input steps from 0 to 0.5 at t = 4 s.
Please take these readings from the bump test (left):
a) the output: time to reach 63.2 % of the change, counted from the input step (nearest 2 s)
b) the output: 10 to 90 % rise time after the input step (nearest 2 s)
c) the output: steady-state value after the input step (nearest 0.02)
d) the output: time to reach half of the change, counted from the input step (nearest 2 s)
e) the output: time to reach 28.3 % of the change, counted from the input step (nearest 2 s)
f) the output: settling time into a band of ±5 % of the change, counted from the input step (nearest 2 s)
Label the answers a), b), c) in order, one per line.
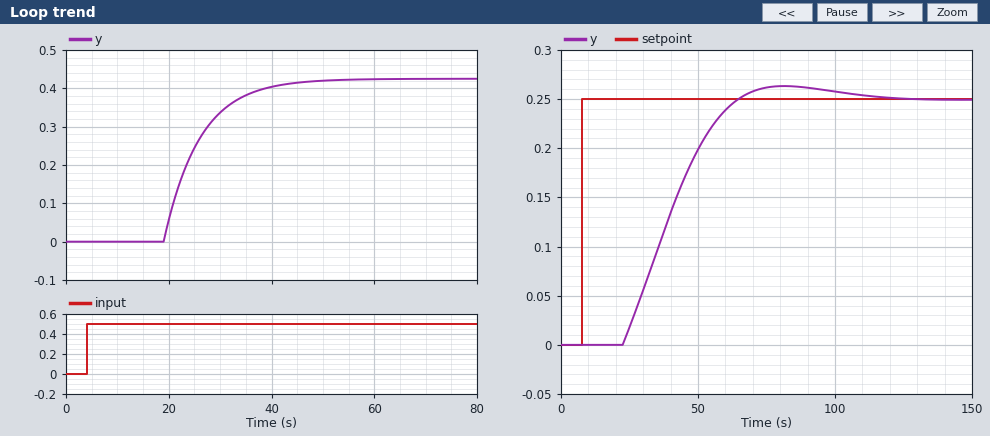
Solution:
a) 22 s
b) 16 s
c) 0.42
d) 20 s
e) 18 s
f) 36 s
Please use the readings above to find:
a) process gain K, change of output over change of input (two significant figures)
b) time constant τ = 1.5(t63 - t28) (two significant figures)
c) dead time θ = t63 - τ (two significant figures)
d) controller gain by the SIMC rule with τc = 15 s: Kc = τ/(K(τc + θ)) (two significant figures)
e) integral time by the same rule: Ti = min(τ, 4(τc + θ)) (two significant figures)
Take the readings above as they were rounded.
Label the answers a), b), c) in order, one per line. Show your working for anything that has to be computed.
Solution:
a) (0.42 - 0) / 0.5 = 0.84
b) 1.5 × (22 - 18) = 6.0 s
c) 22 - 6 = 16 s
d) 6 / (0.84 × (15 + 16)) = 0.23
e) min(6, 4 × (15 + 16)) = 6.0 s
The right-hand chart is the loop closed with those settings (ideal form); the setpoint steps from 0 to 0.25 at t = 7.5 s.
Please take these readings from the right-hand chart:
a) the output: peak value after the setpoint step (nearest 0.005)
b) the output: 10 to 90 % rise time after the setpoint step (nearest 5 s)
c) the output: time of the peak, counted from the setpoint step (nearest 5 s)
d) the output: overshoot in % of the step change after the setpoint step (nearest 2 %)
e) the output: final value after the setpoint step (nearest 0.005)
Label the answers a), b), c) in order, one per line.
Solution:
a) 0.265
b) 30 s
c) 75 s
d) 6 %
e) 0.250
